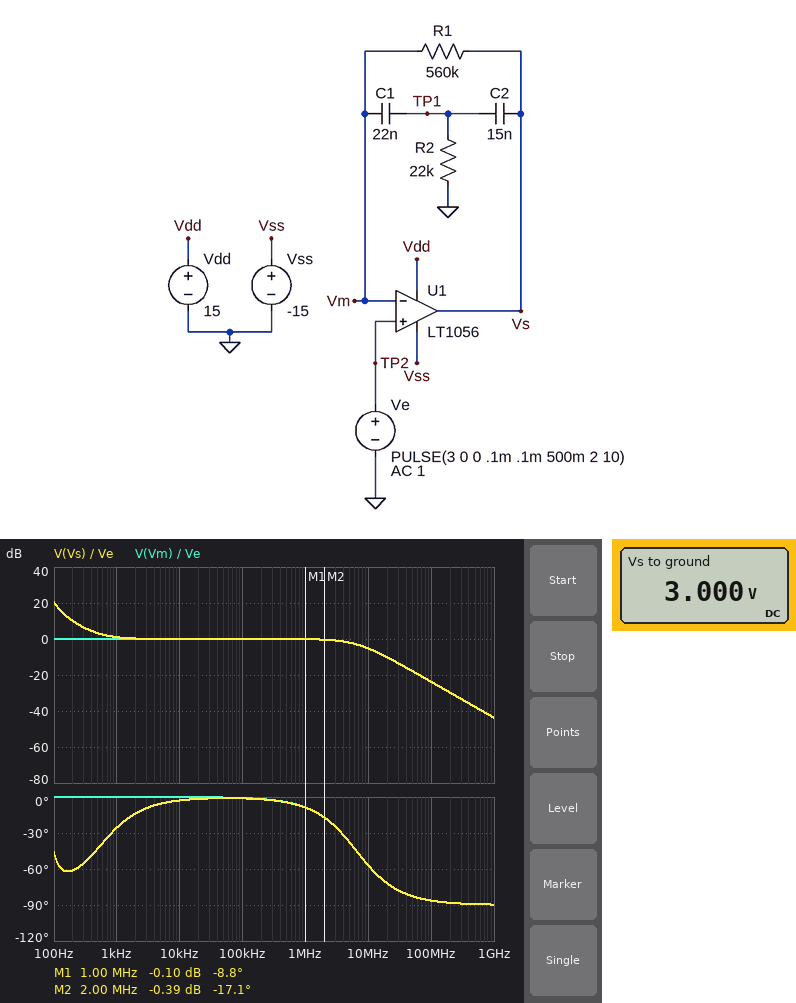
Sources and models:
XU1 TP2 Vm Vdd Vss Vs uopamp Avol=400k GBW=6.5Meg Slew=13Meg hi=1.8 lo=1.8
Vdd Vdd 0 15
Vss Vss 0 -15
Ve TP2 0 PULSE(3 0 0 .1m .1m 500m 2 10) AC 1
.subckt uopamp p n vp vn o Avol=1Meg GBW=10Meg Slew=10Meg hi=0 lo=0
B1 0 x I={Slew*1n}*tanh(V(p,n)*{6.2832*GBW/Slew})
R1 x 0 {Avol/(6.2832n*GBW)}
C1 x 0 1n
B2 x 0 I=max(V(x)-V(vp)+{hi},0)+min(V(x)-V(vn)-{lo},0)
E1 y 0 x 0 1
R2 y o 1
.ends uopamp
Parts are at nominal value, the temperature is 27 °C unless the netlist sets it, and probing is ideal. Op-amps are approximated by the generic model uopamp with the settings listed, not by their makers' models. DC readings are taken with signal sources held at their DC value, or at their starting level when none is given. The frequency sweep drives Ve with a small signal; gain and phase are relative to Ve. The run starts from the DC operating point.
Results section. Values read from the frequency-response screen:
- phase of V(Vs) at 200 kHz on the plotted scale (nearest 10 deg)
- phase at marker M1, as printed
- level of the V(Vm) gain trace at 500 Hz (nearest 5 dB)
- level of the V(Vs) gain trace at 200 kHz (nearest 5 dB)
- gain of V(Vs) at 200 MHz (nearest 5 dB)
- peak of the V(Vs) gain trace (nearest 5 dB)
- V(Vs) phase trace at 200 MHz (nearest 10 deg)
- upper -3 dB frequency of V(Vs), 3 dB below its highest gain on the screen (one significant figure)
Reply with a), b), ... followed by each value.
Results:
a) 0 deg
b) -8.8 deg
c) 0 dB
d) 0 dB
e) -30 dB
f) 20 dB
g) -90 deg
h) 100 Hz
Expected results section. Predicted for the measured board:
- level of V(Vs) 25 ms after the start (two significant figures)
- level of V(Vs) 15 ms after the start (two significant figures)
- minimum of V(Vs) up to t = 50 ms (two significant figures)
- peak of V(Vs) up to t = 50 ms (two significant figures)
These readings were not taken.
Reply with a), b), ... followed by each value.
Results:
a) 670 mV
b) -3.3 V
c) -13 V
d) 7.0 V
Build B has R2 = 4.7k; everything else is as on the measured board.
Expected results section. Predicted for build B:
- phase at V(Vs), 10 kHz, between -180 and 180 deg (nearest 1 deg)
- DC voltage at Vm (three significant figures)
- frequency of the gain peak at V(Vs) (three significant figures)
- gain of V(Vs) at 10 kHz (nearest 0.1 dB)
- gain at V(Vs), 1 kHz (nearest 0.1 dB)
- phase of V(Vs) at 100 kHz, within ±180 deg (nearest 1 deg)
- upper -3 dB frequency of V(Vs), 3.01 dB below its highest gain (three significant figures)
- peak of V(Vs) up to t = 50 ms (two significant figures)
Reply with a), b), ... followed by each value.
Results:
a) -13 deg
b) 3.00 V
c) 171 Hz
d) 0.2 dB
e) 8.2 dB
f) -2 deg
g) 187 Hz
h) 9.9 V
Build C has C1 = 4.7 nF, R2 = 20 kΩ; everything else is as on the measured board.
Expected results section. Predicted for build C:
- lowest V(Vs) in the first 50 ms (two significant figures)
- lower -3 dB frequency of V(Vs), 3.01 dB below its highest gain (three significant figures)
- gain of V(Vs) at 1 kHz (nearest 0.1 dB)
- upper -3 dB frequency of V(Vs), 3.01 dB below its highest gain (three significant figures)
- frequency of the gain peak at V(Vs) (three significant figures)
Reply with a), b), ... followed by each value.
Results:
a) -6.5 V
b) 143 Hz
c) 1.4 dB
d) 224 Hz
e) 179 Hz
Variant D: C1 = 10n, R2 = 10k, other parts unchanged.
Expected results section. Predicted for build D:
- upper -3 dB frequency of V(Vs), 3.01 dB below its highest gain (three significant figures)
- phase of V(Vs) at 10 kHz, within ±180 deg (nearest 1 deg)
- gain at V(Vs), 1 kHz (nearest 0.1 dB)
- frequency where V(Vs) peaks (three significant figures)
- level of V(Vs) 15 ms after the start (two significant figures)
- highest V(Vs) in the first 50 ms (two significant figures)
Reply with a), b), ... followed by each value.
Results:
a) 199 Hz
b) -6 deg
c) 3.6 dB
d) 174 Hz
e) 680 mV
f) 8.7 V
